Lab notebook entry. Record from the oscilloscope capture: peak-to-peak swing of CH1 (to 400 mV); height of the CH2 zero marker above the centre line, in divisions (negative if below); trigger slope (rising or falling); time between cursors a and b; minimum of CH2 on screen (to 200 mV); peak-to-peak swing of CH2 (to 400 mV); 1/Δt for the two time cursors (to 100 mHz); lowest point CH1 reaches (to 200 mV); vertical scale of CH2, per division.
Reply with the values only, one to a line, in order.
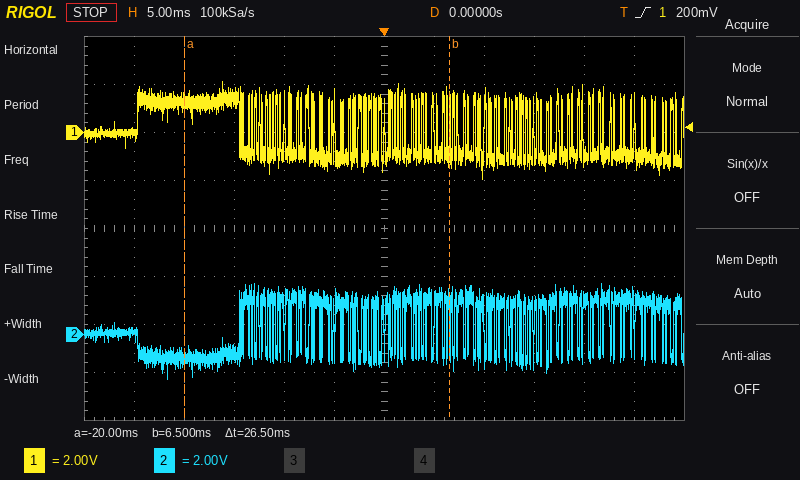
4.0 V
-2.2 div
rising
26.5 ms
-1.8 V
4.0 V
37.7 Hz
-2.0 V
2 V
